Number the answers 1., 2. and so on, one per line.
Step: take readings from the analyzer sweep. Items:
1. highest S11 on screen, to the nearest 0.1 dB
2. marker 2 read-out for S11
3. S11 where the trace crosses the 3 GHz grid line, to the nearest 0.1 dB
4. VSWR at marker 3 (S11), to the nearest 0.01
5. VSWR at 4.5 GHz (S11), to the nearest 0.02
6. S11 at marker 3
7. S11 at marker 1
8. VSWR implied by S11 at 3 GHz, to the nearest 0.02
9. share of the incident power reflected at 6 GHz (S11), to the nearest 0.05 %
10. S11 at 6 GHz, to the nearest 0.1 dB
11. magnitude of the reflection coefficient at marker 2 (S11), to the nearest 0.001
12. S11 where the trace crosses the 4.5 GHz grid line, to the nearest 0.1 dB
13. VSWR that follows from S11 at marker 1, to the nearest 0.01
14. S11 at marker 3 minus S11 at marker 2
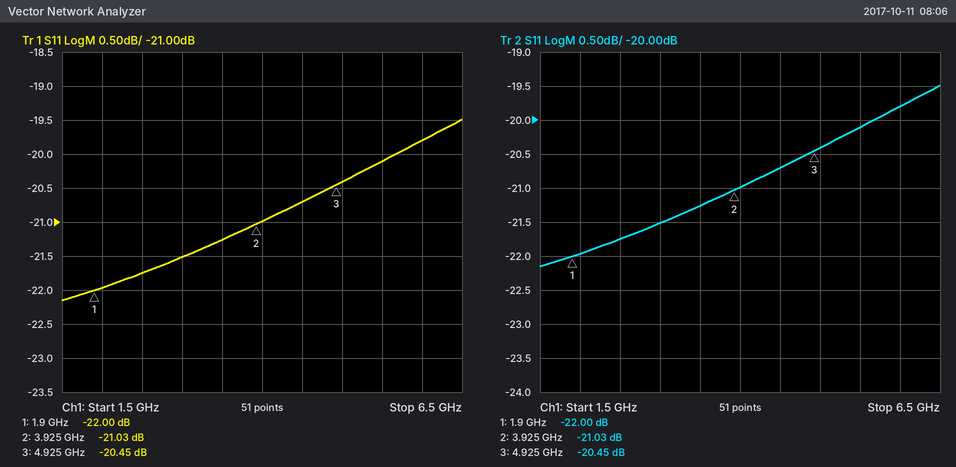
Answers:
1. -19.5 dB
2. -21.03 dB
3. -21.5 dB
4. 1.21
5. 1.20
6. -20.45 dB
7. -22.00 dB
8. 1.18
9. 1.05 %
10. -19.8 dB
11. 0.089
12. -20.7 dB
13. 1.17
14. 0.58 dB
